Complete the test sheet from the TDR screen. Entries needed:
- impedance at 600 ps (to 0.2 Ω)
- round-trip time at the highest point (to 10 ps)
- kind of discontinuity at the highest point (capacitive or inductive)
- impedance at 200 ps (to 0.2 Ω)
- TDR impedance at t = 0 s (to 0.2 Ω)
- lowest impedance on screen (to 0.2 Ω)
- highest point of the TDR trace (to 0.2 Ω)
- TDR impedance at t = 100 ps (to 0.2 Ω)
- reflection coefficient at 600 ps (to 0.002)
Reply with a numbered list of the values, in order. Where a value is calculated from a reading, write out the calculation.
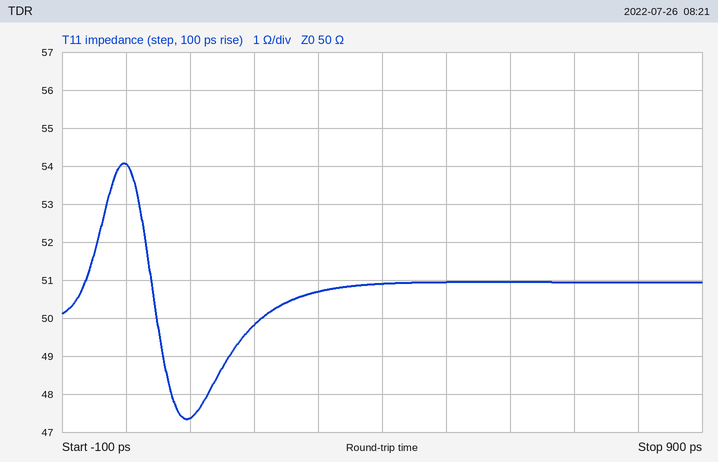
1. 51.0 Ω
2. 0 ps
3. inductive
4. 49.8 Ω
5. 54.0 Ω
6. 47.4 Ω
7. 54.0 Ω
8. 47.4 Ω
9. (51 − 50)/(51 + 50) ≈ +0.010
